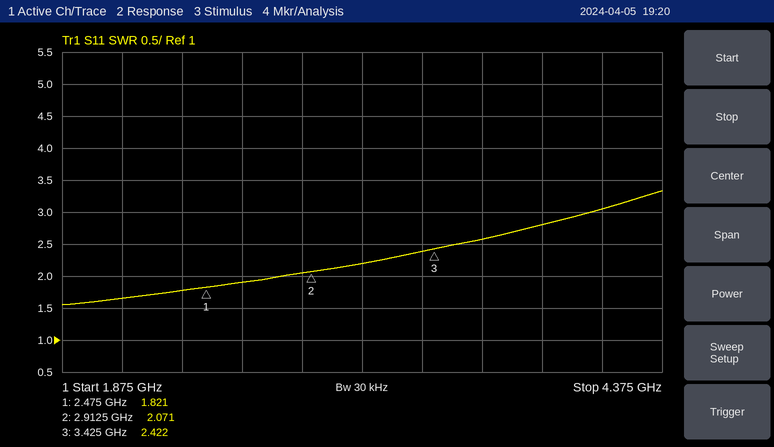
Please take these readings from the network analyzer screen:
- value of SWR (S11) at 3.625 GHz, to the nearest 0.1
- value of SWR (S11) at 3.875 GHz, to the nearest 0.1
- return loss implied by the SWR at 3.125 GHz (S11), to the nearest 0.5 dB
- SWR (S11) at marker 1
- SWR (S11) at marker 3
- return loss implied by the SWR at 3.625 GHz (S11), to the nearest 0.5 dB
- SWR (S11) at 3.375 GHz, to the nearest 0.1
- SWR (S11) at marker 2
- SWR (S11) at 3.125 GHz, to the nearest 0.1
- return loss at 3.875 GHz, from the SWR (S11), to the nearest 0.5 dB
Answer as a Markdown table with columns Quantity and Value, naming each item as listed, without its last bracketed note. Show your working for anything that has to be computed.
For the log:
| Quantity | Value |
|---|---|
| value of SWR (S11) at 3.625 GHz, to the nearest 0.1 | 2.6 |
| value of SWR (S11) at 3.875 GHz, to the nearest 0.1 | 2.8 |
| return loss implied by the SWR at 3.125 GHz (S11), to the nearest 0.5 dB | −20 log10((2.2 − 1)/(2.2 + 1)) ≈ 8.5 dB |
| SWR (S11) at marker 1 | 1.821 |
| SWR (S11) at marker 3 | 2.422 |
| return loss implied by the SWR at 3.625 GHz (S11), to the nearest 0.5 dB | −20 log10((2.6 − 1)/(2.6 + 1)) ≈ 7.0 dB |
| SWR (S11) at 3.375 GHz, to the nearest 0.1 | 2.4 |
| SWR (S11) at marker 2 | 2.071 |
| SWR (S11) at 3.125 GHz, to the nearest 0.1 | 2.2 |
| return loss at 3.875 GHz, from the SWR (S11), to the nearest 0.5 dB | −20 log10((2.8 − 1)/(2.8 + 1)) ≈ 6.5 dB |
